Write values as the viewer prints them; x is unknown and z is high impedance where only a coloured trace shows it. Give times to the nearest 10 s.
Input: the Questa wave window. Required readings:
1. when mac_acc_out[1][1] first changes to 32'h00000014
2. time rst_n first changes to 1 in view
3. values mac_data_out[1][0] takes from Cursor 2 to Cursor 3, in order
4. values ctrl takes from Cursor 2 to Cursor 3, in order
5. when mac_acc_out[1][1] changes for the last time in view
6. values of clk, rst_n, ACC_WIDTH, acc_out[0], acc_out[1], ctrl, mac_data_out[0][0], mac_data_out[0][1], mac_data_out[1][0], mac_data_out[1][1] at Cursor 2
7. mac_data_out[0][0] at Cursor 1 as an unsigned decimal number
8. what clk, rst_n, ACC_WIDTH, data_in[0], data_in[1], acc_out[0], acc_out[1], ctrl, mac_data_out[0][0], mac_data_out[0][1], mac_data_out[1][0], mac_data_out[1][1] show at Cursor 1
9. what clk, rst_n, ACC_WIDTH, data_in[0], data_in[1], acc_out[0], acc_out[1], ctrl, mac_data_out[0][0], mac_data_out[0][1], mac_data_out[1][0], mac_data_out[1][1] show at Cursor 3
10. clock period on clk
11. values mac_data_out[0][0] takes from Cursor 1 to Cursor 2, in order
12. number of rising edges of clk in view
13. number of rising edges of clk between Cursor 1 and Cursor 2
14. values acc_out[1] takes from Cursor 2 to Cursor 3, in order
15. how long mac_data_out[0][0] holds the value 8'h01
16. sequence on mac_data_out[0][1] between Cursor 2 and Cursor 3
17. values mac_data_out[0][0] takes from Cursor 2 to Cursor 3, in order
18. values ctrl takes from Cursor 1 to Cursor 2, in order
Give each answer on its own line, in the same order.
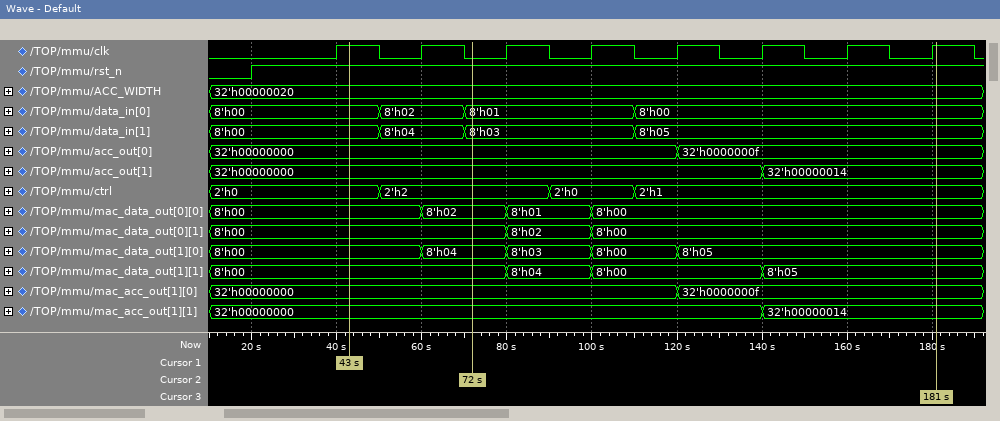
140 s
20 s
8'h04, 8'h03, 8'h00, 8'h05
2'h2, 2'h0, 2'h1
140 s
clk=0, rst_n=1, ACC_WIDTH=32'h00000020, acc_out[0]=32'h00000000, acc_out[1]=32'h00000000, ctrl=2'h2, mac_data_out[0][0]=8'h02, mac_data_out[0][1]=8'h00, mac_data_out[1][0]=8'h04, mac_data_out[1][1]=8'h00
0
clk=1, rst_n=1, ACC_WIDTH=32'h00000020, data_in[0]=8'h00, data_in[1]=8'h00, acc_out[0]=32'h00000000, acc_out[1]=32'h00000000, ctrl=2'h0, mac_data_out[0][0]=8'h00, mac_data_out[0][1]=8'h00, mac_data_out[1][0]=8'h00, mac_data_out[1][1]=8'h00
clk=1, rst_n=1, ACC_WIDTH=32'h00000020, data_in[0]=8'h00, data_in[1]=8'h05, acc_out[0]=32'h0000000f, acc_out[1]=32'h00000014, ctrl=2'h1, mac_data_out[0][0]=8'h00, mac_data_out[0][1]=8'h00, mac_data_out[1][0]=8'h05, mac_data_out[1][1]=8'h05
20 s
8'h00, 8'h02
8
1
32'h00000000, 32'h00000014
20 s
8'h00, 8'h02, 8'h00
8'h02, 8'h01, 8'h00
2'h0, 2'h2
